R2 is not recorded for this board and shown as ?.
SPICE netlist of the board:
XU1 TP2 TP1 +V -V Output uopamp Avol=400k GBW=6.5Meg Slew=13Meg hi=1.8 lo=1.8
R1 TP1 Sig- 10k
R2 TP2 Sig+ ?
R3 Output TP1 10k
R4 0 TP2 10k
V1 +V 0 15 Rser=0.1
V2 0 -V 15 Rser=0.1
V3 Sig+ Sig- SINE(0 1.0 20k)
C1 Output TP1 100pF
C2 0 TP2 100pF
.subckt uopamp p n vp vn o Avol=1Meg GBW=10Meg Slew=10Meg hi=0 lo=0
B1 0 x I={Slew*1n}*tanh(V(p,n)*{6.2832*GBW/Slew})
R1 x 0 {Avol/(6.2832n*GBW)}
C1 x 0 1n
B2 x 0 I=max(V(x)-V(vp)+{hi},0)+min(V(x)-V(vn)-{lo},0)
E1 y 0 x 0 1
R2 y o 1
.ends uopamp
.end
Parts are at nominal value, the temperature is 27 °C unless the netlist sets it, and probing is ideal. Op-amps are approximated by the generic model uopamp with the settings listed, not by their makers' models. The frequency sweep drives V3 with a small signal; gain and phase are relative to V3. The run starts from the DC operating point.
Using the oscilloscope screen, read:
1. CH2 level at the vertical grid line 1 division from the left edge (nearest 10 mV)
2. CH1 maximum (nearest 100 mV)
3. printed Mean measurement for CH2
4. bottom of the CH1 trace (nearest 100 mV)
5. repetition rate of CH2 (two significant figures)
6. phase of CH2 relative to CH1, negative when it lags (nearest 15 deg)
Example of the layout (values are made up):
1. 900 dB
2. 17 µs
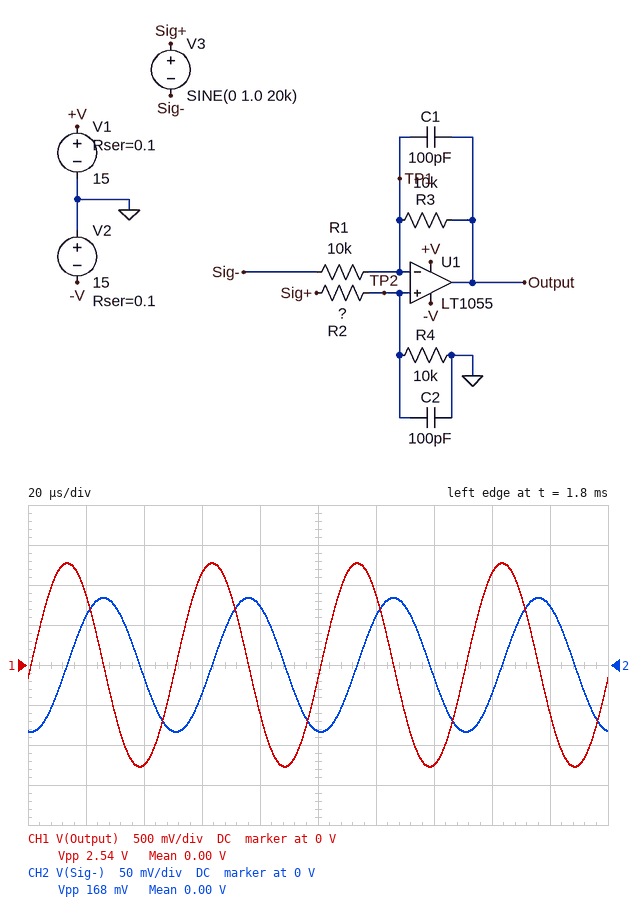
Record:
1. 60 mV
2. 1.3 V
3. 0.00 V
4. -1.3 V
5. 20 kHz
6. -90 deg
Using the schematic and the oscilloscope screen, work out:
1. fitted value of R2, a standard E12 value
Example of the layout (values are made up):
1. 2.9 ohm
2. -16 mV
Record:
1. 5.6 kΩ
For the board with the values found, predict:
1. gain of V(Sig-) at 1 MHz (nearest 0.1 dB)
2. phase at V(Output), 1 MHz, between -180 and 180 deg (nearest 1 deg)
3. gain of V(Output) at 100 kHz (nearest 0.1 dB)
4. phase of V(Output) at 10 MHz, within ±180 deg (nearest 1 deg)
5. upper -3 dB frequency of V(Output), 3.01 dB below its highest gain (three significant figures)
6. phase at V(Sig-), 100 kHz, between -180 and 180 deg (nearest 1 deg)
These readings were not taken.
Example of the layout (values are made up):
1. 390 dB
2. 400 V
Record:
1. -3.8 dB
2. -90 deg
3. 0.6 dB
4. -145 deg
5. 154 kHz
6. -123 deg
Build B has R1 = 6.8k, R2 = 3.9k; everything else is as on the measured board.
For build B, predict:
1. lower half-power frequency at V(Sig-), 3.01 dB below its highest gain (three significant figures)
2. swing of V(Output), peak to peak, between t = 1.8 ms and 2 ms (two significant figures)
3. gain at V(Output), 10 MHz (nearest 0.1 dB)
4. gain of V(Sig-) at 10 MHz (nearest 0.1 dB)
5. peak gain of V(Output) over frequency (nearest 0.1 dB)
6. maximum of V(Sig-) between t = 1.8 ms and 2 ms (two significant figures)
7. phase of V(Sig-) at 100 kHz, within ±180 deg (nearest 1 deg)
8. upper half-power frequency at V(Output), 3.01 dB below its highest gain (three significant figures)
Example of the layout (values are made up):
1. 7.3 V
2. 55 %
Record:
1. 114 kHz
2. 3.7 V
3. -35.9 dB
4. -3.9 dB
5. 5.4 dB
6. 310 mV
7. -88 deg
8. 152 kHz
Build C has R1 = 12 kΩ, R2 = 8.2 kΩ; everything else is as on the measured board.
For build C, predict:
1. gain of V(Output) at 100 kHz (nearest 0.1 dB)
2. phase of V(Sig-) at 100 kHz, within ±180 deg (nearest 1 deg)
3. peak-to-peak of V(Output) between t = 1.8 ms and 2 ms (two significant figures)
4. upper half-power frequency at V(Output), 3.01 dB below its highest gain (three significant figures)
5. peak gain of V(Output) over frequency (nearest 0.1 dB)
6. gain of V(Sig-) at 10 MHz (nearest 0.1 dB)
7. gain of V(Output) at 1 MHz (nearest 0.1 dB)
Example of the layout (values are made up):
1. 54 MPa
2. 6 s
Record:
1. -1.6 dB
2. -137 deg
3. 2.0 V
4. 155 kHz
5. -0.1 dB
6. -4.5 dB
7. -16.5 dB
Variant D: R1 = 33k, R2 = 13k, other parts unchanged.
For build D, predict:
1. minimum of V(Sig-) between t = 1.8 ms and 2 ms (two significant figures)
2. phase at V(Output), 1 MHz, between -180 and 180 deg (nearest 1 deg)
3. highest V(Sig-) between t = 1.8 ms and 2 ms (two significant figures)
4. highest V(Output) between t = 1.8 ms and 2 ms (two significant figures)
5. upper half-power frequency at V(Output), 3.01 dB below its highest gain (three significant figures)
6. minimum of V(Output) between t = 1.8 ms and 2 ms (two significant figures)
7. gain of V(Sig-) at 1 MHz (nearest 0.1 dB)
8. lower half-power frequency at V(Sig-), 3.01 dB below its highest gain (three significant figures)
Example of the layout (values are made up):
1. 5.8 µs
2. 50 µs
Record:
1. -500 mV
2. -90 deg
3. 500 mV
4. 430 mV
5. 157 kHz
6. -430 mV
7. -2.9 dB
8. 28.8 kHz
